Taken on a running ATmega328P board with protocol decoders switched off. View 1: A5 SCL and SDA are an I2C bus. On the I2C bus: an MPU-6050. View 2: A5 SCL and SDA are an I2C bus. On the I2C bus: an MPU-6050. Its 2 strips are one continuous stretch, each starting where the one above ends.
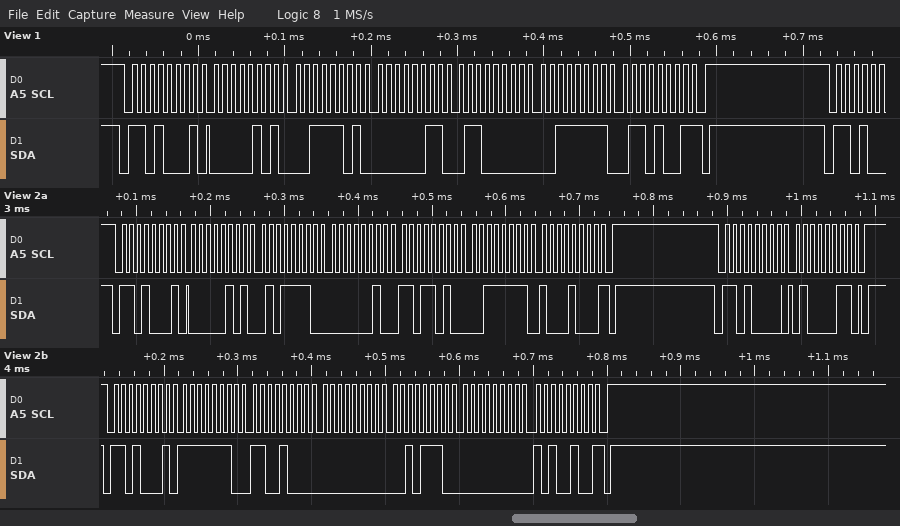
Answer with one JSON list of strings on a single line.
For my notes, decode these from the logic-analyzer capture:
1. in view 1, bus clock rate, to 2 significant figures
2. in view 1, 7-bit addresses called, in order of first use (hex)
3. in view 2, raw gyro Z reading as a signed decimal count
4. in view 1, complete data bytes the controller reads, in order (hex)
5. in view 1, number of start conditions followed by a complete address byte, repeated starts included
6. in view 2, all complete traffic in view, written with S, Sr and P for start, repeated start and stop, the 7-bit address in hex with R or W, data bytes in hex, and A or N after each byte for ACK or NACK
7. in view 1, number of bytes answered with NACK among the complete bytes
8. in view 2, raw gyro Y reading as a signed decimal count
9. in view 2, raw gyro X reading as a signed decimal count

["100 kHz", "0x68", "164", "05 3D 03 60 3F 69", "1", "S 68R A 05 A 5E A 02 A DA A 3F A 88 N P S 68W A 43 A P S 68R A FE A C8 A 00 A 2E A 00 A A4 N P", "1", "46", "-312"]
